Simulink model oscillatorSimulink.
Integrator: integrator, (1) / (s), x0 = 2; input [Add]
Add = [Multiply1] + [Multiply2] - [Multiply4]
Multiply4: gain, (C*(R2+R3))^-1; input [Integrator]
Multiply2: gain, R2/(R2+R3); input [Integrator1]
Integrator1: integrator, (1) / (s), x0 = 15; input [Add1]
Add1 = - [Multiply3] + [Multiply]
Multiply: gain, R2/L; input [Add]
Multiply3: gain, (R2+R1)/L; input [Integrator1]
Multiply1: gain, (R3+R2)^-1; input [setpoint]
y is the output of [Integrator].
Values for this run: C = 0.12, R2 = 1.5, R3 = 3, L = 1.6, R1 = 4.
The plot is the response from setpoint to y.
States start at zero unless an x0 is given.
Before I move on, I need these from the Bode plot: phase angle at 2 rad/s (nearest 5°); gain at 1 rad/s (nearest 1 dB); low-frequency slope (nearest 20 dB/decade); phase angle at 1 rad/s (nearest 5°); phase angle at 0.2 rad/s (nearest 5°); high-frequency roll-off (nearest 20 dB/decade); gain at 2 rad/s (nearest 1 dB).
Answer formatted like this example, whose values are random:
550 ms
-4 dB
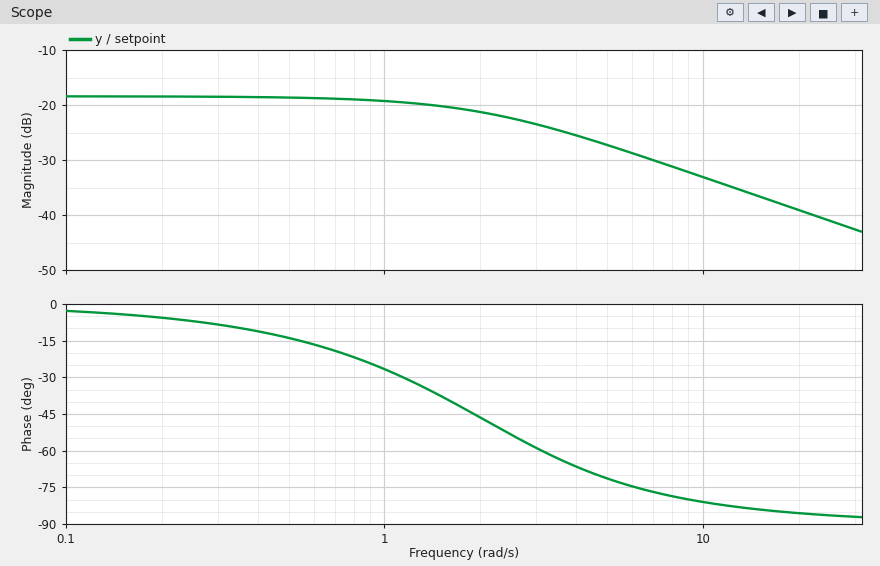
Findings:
-45°
-19 dB
0 dB/decade
-25°
-5°
-20 dB/decade
-21 dB
